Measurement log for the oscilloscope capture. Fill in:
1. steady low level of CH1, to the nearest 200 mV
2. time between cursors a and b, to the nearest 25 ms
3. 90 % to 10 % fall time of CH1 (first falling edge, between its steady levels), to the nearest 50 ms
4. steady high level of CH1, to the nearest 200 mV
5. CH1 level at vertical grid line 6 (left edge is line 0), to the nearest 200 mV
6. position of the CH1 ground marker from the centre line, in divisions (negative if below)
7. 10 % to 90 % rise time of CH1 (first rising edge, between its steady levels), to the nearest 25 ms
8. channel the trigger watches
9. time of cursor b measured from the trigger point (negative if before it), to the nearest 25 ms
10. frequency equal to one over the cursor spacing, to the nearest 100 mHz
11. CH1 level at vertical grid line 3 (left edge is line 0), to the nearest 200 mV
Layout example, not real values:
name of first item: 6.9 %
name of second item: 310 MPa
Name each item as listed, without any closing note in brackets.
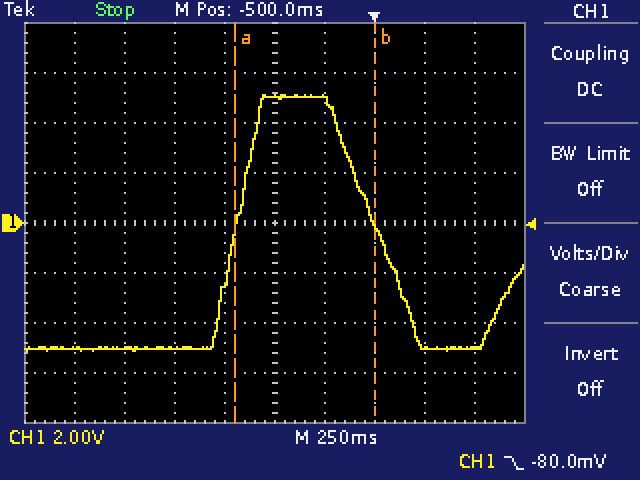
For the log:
steady low level of CH1, to the nearest 200 mV: -5.0 V
time between cursors a and b, to the nearest 25 ms: 700 ms
90 % to 10 % fall time of CH1 (first falling edge, between its steady levels), to the nearest 50 ms: 400 ms
steady high level of CH1, to the nearest 200 mV: 5.0 V
CH1 level at vertical grid line 6 (left edge is line 0), to the nearest 200 mV: 5.0 V
position of the CH1 ground marker from the centre line, in divisions: 0.0 div
10 % to 90 % rise time of CH1 (first rising edge, between its steady levels), to the nearest 25 ms: 200 ms
channel the trigger watches: CH1
time of cursor b measured from the trigger point (negative if before it), to the nearest 25 ms: 0 ms
frequency equal to one over the cursor spacing, to the nearest 100 mHz: 1.4 Hz
CH1 level at vertical grid line 3 (left edge is line 0), to the nearest 200 mV: -5.0 V
